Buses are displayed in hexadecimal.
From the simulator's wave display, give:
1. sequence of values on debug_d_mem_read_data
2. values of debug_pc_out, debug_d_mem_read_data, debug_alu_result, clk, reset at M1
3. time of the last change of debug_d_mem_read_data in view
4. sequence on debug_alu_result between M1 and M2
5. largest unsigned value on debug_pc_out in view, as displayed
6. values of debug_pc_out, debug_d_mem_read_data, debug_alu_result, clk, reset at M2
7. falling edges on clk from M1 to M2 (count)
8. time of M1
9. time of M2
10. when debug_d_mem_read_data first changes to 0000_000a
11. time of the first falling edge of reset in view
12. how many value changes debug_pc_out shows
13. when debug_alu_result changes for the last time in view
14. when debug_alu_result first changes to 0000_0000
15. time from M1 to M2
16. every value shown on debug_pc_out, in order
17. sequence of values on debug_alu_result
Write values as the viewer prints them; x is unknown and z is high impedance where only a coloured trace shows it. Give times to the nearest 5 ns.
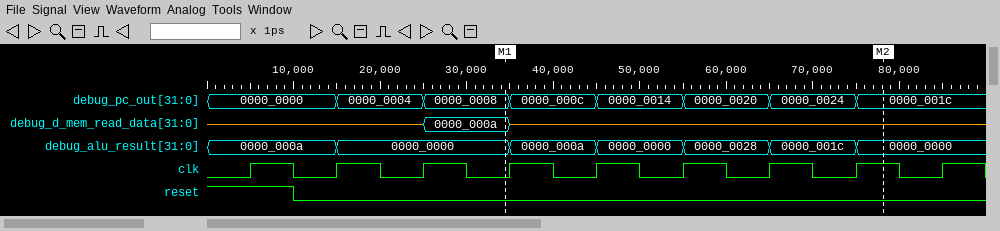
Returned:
z, 0000_000a, z
debug_pc_out=0000_0008, debug_d_mem_read_data=0000_000a, debug_alu_result=0000_0000, clk=0, reset=0
35 ns
0000_0000, 0000_000a, 0000_0000, 0000_0028, 0000_001c, 0000_0000
0000_0024
debug_pc_out=0000_001c, debug_d_mem_read_data=z, debug_alu_result=0000_0000, clk=1, reset=0
4
35 ns
80 ns
25 ns
10 ns
7
75 ns
15 ns
45 ns
0000_0000, 0000_0004, 0000_0008, 0000_000c, 0000_0014, 0000_0020, 0000_0024, 0000_001c
0000_000a, 0000_0000, 0000_000a, 0000_0000, 0000_0028, 0000_001c, 0000_0000
